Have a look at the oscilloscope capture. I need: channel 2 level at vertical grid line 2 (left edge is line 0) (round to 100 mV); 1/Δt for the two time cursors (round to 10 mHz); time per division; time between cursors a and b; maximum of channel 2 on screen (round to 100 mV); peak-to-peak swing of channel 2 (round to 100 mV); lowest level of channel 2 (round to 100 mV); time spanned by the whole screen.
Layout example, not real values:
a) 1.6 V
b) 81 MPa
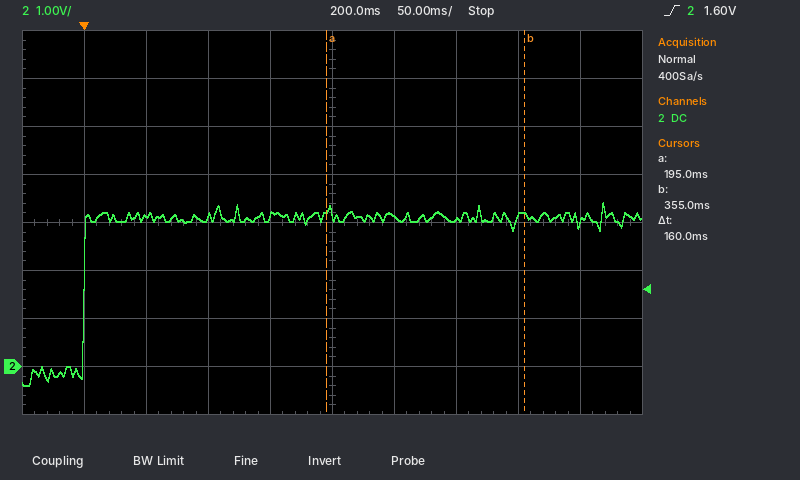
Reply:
a) 3.1 V
b) 6.25 Hz
c) 50 ms
d) 160 ms
e) 3.4 V
f) 3.8 V
g) -400 mV
h) 500 ms
